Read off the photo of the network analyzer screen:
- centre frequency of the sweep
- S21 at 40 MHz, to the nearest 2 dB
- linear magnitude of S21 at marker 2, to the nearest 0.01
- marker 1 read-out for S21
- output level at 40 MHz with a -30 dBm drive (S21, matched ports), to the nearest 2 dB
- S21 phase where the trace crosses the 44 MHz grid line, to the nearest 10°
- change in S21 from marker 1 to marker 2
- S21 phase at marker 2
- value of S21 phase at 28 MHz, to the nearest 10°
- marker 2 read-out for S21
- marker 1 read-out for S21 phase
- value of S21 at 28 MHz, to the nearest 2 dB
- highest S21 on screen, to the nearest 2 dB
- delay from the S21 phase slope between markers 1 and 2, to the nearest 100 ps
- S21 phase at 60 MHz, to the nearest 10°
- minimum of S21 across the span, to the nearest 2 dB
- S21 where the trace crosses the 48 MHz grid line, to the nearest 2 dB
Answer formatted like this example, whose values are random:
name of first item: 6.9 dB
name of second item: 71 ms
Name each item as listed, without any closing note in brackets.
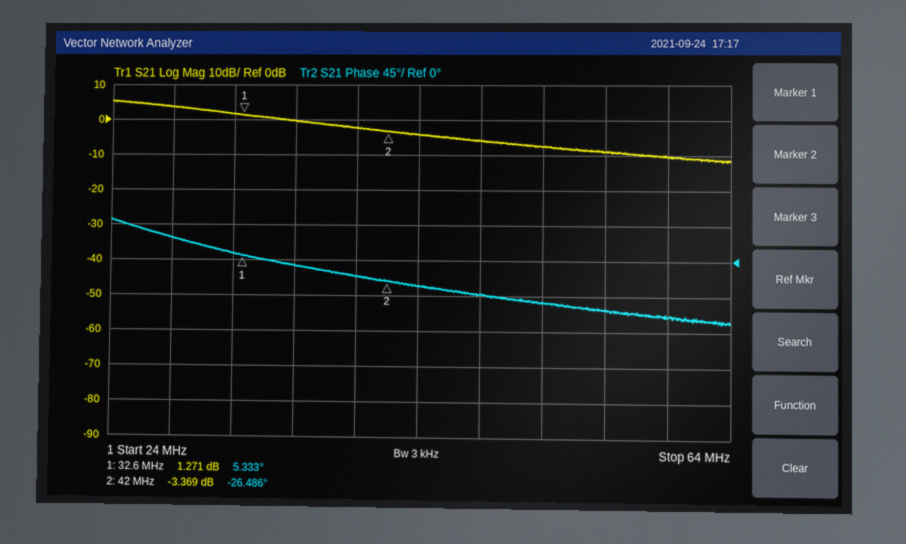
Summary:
centre frequency of the sweep: 44 MHz
S21 at 40 MHz, to the nearest 2 dB: -2 dB
linear magnitude of S21 at marker 2, to the nearest 0.01: 0.68
marker 1 read-out for S21: 1.271 dB
output level at 40 MHz with a -30 dBm drive (S21, matched ports), to the nearest 2 dB: -32 dBm
S21 phase where the trace crosses the 44 MHz grid line, to the nearest 10°: -30°
change in S21 from marker 1 to marker 2: -4.640 dB
S21 phase at marker 2: -26.486°
value of S21 phase at 28 MHz, to the nearest 10°: 30°
marker 2 read-out for S21: -3.369 dB
marker 1 read-out for S21 phase: 5.333°
value of S21 at 28 MHz, to the nearest 2 dB: 4 dB
highest S21 on screen, to the nearest 2 dB: 6 dB
delay from the S21 phase slope between markers 1 and 2, to the nearest 100 ps: 9.4 ns
S21 phase at 60 MHz, to the nearest 10°: -70°
minimum of S21 across the span, to the nearest 2 dB: -12 dB
S21 where the trace crosses the 48 MHz grid line, to the nearest 2 dB: -6 dB
